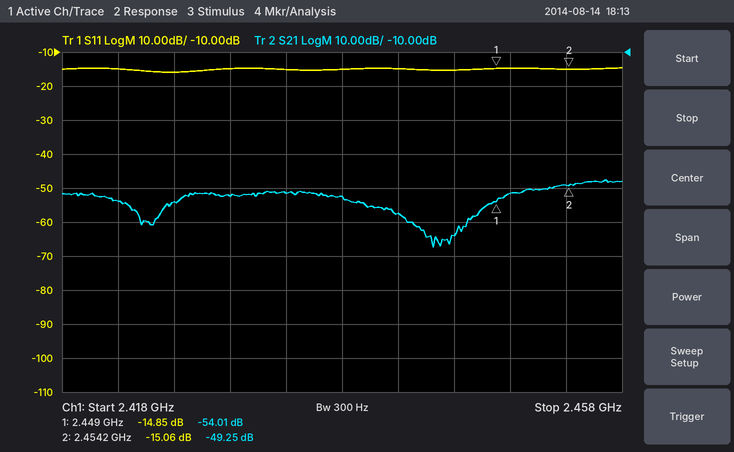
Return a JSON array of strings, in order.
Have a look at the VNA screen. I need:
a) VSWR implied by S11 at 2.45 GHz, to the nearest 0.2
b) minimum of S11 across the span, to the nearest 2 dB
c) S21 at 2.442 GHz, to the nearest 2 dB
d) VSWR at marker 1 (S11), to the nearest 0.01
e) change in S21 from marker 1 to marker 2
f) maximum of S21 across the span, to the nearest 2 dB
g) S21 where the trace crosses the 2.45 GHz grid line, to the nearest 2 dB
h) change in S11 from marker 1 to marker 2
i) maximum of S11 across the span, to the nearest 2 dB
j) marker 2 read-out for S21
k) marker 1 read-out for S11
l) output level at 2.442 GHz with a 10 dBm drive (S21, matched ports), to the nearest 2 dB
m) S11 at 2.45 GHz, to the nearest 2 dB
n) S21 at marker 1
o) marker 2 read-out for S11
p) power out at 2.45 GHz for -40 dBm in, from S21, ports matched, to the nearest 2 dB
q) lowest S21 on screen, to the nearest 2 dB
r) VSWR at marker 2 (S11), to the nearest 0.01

["1.4", "-16 dB", "-58 dB", "1.44", "4.76 dB", "-48 dB", "-52 dB", "-0.21 dB", "-14 dB", "-49.25 dB", "-14.85 dB", "-48 dBm", "-14 dB", "-54.01 dB", "-15.06 dB", "-92 dBm", "-68 dB", "1.43"]
